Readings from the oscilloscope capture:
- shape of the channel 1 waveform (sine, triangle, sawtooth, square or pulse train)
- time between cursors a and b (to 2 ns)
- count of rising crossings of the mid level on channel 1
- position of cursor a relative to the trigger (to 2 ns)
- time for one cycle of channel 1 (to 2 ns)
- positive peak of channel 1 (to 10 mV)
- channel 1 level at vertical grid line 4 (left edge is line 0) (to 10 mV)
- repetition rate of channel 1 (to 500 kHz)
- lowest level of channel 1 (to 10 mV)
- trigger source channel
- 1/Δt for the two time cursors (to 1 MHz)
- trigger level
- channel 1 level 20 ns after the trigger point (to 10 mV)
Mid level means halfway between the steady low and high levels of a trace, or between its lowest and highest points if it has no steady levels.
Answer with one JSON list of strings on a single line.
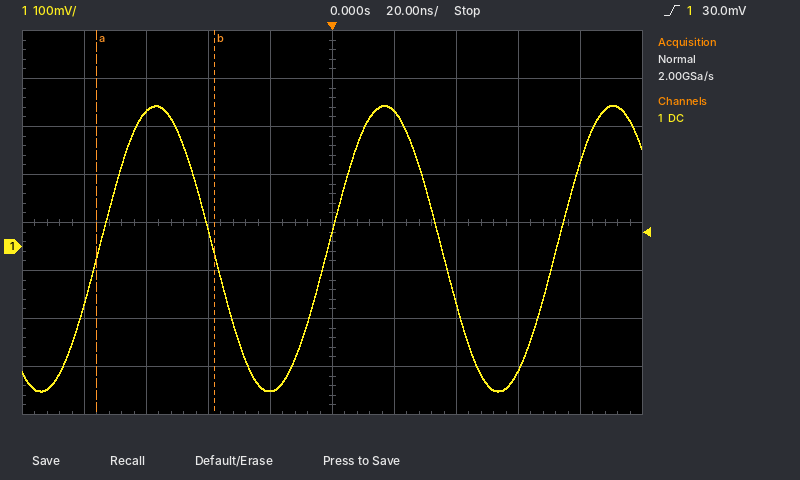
["sine", "38 ns", "3", "-76 ns", "74 ns", "290 mV", "-300 mV", "13.5 MHz", "-300 mV", "channel 1", "26 MHz", "30.0 mV", "280 mV"]
